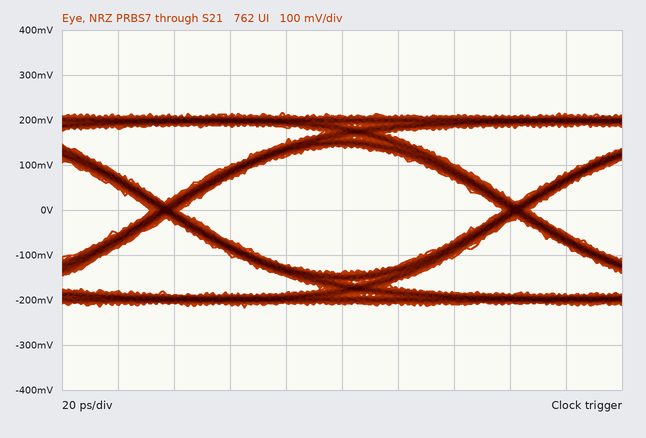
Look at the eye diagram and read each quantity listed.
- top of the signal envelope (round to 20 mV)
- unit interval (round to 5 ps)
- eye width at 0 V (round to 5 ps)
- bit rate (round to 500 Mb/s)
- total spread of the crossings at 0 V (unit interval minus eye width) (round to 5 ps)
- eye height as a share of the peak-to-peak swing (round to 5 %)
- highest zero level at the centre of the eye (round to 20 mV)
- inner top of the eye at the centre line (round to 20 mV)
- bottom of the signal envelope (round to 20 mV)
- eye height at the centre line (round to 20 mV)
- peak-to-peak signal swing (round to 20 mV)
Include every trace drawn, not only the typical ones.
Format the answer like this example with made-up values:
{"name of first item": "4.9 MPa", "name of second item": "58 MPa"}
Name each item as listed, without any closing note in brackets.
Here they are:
{"top of the signal envelope": "220 mV", "unit interval": "125 ps", "eye width at 0 V": "115 ps", "bit rate": "8.0 Gb/s", "total spread of the crossings at 0 V (unit interval minus eye width)": "10 ps", "eye height as a share of the peak-to-peak swing": "65 %", "highest zero level at the centre of the eye": "-140 mV", "inner top of the eye at the centre line": "140 mV", "bottom of the signal envelope": "-220 mV", "eye height at the centre line": "280 mV", "peak-to-peak signal swing": "440 mV"}
